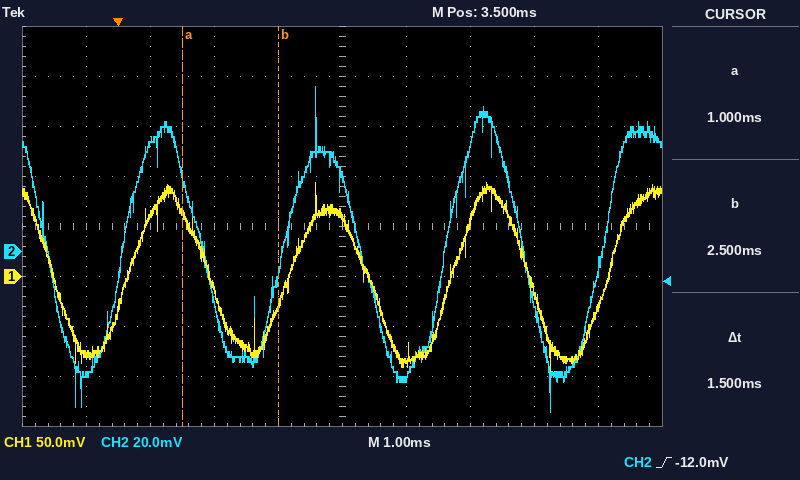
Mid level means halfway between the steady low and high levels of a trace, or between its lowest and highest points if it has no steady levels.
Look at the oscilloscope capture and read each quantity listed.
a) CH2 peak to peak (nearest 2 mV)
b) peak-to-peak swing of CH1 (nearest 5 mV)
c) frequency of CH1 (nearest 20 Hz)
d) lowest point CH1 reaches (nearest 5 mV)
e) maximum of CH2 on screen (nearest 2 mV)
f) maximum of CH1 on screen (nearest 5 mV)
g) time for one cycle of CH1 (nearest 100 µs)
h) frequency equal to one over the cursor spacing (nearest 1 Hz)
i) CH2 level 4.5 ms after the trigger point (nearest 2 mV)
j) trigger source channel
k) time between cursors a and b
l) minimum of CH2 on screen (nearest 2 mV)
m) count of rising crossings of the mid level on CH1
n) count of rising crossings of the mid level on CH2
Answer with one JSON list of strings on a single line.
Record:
["130 mV", "190 mV", "400 Hz", "-95 mV", "66 mV", "95 mV", "2.5 ms", "667 Hz", "-50 mV", "CH2", "1.5 ms", "-64 mV", "4", "4"]
